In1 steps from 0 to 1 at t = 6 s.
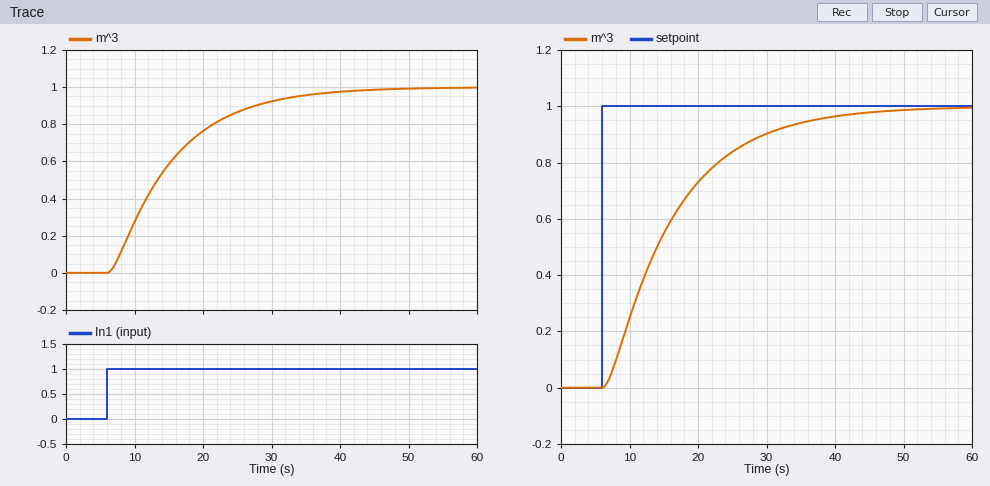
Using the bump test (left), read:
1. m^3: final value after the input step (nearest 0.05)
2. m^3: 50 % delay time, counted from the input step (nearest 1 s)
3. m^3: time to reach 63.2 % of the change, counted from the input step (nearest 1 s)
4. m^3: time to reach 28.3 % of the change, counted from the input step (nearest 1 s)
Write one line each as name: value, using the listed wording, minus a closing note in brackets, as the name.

m^3: final value after the input step: 1.00
m^3: 50 % delay time, counted from the input step: 7 s
m^3: time to reach 63.2 % of the change, counted from the input step: 10 s
m^3: time to reach 28.3 % of the change, counted from the input step: 4 s
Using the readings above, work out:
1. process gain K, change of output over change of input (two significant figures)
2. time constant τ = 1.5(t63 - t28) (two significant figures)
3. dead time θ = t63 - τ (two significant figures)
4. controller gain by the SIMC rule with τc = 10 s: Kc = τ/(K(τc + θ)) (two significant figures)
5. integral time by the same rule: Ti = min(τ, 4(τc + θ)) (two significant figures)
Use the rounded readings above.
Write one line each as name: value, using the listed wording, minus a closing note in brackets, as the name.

process gain K, change of output over change of input: 1.0
time constant τ = 1.5(t63 - t28): 9.0 s
dead time θ = t63 - τ: 1.0 s
controller gain by the SIMC rule with τc = 10 s: Kc = τ/(K(τc + θ)): 0.82
integral time by the same rule: Ti = min(τ, 4(τc + θ)): 9.0 s
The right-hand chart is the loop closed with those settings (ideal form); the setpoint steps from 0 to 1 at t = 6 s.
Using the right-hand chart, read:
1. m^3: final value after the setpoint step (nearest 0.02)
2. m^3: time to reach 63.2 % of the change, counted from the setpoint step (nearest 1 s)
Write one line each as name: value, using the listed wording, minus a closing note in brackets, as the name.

m^3: final value after the setpoint step: 1.00
m^3: time to reach 63.2 % of the change, counted from the setpoint step: 11 s
